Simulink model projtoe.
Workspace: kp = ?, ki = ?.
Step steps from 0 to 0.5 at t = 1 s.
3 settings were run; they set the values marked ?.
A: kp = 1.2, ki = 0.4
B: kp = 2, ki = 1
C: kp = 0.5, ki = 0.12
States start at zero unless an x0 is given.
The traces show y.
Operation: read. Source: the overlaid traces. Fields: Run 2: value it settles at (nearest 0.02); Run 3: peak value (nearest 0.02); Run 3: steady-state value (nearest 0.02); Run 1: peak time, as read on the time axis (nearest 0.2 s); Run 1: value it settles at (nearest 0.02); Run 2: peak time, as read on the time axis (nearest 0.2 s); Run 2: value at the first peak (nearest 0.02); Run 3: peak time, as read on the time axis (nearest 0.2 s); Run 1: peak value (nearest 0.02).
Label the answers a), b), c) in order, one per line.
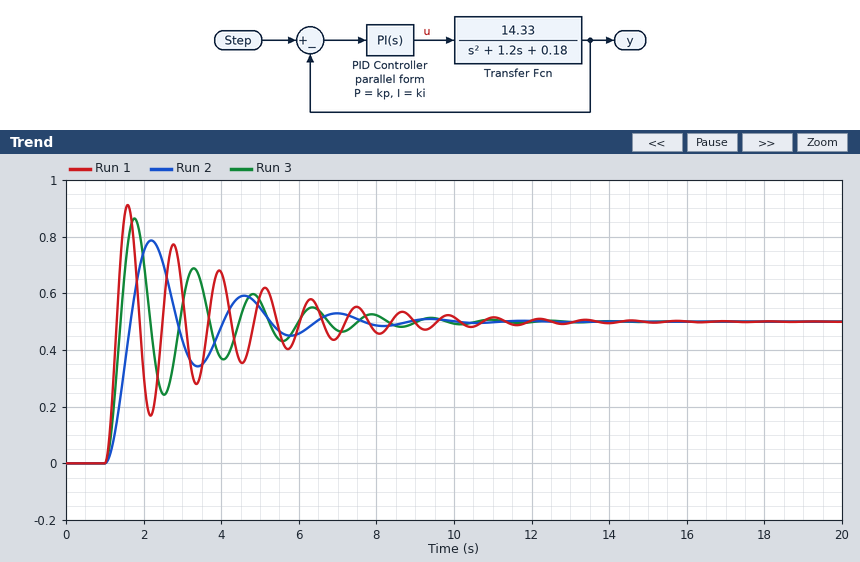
a) 0.50
b) 0.86
c) 0.50
d) 1.6 s
e) 0.50
f) 2.2 s
g) 0.78
h) 1.8 s
i) 0.92
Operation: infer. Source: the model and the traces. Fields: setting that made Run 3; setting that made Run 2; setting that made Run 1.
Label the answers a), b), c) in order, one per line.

a) A
b) C
c) B
